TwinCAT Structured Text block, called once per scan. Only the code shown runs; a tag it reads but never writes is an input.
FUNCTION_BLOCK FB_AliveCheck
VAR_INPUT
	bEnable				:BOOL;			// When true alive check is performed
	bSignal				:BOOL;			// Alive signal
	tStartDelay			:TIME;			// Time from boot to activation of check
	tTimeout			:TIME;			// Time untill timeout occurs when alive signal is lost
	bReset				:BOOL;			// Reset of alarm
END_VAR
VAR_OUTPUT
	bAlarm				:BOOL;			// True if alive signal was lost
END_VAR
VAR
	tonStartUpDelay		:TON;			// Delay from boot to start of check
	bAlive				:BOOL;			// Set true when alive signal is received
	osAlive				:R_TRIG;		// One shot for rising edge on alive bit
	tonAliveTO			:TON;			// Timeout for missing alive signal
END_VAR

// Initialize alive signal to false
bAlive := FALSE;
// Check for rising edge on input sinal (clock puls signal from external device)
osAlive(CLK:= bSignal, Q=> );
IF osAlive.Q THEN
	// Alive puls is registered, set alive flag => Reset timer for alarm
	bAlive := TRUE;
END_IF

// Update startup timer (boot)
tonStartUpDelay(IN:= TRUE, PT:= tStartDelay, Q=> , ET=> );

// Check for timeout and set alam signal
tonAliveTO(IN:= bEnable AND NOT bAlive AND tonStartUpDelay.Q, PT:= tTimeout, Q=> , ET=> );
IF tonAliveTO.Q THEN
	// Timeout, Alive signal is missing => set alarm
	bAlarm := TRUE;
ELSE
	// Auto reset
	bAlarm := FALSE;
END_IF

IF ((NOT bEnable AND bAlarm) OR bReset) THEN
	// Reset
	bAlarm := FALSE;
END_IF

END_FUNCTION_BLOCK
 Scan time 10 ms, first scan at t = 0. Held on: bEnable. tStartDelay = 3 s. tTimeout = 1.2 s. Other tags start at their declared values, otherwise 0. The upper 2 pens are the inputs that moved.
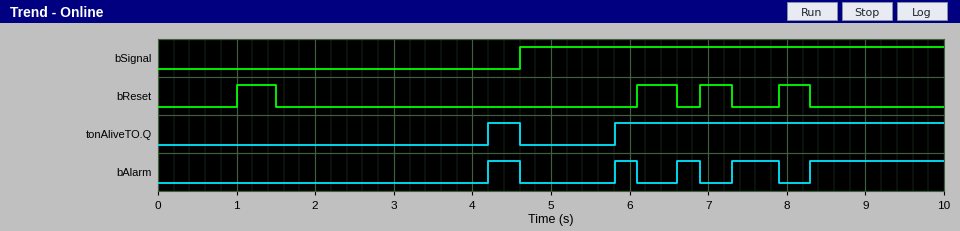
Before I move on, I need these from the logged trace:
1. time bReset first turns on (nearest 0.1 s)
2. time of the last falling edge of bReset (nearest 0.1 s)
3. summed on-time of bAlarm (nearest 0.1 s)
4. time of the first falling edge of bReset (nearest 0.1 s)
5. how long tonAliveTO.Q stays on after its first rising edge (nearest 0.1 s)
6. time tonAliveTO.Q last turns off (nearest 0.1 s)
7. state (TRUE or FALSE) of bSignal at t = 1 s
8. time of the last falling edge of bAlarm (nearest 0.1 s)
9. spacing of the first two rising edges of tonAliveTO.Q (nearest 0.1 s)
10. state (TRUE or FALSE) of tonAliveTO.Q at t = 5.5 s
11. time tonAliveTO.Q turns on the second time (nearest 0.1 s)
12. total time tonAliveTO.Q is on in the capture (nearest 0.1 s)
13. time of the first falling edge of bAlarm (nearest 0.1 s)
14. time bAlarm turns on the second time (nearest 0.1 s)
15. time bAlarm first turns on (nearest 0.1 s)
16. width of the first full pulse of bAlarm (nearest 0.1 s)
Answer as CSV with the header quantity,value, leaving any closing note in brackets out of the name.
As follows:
quantity,value
time bReset first turns on,1.0 s
time of the last falling edge of bReset,8.3 s
summed on-time of bAlarm,3.3 s
time of the first falling edge of bReset,1.5 s
how long tonAliveTO.Q stays on after its first rising edge,0.4 s
time tonAliveTO.Q last turns off,4.6 s
state (TRUE or FALSE) of bSignal at t = 1 s,FALSE
time of the last falling edge of bAlarm,7.9 s
spacing of the first two rising edges of tonAliveTO.Q,1.6 s
state (TRUE or FALSE) of tonAliveTO.Q at t = 5.5 s,FALSE
time tonAliveTO.Q turns on the second time,5.8 s
total time tonAliveTO.Q is on in the capture,4.6 s
time of the first falling edge of bAlarm,4.6 s
time bAlarm turns on the second time,5.8 s
time bAlarm first turns on,4.2 s
width of the first full pulse of bAlarm,0.4 s
